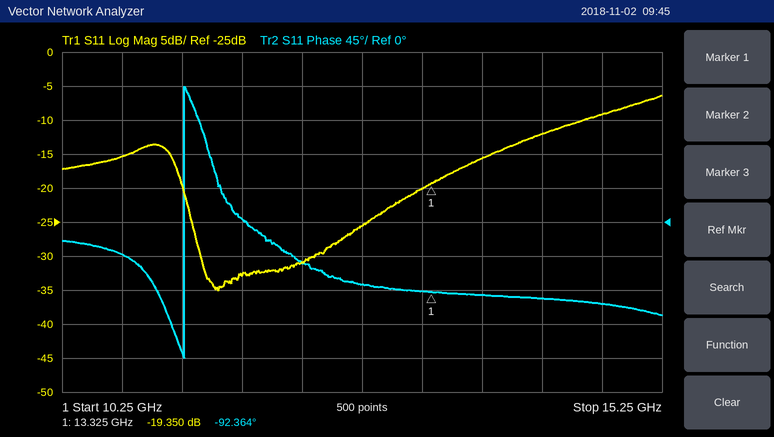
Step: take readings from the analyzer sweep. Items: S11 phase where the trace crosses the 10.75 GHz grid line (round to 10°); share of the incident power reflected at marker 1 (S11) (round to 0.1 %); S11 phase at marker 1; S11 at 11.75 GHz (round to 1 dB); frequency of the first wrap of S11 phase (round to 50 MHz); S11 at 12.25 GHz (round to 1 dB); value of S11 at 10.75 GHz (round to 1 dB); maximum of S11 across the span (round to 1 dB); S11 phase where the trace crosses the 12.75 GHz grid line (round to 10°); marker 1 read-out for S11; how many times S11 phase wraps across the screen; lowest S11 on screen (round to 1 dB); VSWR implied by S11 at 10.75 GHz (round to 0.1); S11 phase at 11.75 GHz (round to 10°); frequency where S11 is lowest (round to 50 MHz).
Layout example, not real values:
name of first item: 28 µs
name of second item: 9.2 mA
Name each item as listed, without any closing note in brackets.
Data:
S11 phase where the trace crosses the 10.75 GHz grid line: -40°
share of the incident power reflected at marker 1 (S11): 1.2 %
S11 phase at marker 1: -92.364°
S11 at 11.75 GHz: -33 dB
frequency of the first wrap of S11 phase: 11.25 GHz
S11 at 12.25 GHz: -31 dB
value of S11 at 10.75 GHz: -15 dB
maximum of S11 across the span: -6 dB
S11 phase where the trace crosses the 12.75 GHz grid line: -80°
marker 1 read-out for S11: -19.350 dB
how many times S11 phase wraps across the screen: 1
lowest S11 on screen: -35 dB
VSWR implied by S11 at 10.75 GHz: 1.4
S11 phase at 11.75 GHz: 0°
frequency where S11 is lowest: 11.55 GHz
